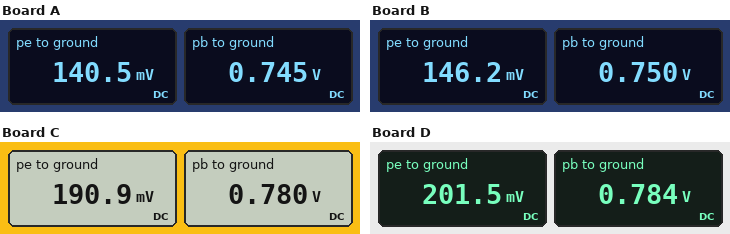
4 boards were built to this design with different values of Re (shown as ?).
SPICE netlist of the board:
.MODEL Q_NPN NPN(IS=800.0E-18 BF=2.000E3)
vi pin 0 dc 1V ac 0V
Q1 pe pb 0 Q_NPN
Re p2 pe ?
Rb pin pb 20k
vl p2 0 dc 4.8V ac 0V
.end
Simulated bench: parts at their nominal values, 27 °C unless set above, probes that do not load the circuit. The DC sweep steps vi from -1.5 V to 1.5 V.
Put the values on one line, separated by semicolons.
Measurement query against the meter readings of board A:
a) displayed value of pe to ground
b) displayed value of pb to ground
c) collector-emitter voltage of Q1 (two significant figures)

140.5 mV; 0.745 V; 140 mV
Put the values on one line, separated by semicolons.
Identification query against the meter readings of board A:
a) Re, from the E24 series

1.8 kΩ
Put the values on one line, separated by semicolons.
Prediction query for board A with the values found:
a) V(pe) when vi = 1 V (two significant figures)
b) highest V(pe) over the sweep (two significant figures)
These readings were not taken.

140 mV; 4.8 V
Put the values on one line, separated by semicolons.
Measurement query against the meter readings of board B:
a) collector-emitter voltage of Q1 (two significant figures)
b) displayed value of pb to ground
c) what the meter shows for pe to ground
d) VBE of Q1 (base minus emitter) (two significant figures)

150 mV; 0.750 V; 146.2 mV; 750 mV
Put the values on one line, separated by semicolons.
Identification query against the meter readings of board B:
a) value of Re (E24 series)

1.5 kΩ
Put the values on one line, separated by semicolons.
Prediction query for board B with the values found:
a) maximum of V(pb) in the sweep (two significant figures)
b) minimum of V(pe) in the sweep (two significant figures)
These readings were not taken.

750 mV; 120 mV
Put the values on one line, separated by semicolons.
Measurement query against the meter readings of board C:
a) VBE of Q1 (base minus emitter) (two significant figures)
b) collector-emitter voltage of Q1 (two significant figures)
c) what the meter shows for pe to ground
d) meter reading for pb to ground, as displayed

780 mV; 190 mV; 190.9 mV; 0.780 V
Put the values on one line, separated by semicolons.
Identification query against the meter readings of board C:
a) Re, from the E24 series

470 Ω
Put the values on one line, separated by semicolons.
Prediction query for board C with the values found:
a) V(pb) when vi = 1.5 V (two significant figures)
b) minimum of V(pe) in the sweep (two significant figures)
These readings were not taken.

780 mV; 150 mV
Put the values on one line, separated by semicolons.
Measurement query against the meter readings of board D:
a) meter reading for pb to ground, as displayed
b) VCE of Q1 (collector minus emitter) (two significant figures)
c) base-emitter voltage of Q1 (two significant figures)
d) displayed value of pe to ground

0.784 V; 200 mV; 780 mV; 201.5 mV
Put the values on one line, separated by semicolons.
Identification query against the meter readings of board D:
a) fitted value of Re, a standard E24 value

390 Ω
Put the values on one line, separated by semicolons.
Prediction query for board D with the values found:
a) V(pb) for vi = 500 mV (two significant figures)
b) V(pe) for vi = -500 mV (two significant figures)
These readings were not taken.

500 mV; 4.8 V
